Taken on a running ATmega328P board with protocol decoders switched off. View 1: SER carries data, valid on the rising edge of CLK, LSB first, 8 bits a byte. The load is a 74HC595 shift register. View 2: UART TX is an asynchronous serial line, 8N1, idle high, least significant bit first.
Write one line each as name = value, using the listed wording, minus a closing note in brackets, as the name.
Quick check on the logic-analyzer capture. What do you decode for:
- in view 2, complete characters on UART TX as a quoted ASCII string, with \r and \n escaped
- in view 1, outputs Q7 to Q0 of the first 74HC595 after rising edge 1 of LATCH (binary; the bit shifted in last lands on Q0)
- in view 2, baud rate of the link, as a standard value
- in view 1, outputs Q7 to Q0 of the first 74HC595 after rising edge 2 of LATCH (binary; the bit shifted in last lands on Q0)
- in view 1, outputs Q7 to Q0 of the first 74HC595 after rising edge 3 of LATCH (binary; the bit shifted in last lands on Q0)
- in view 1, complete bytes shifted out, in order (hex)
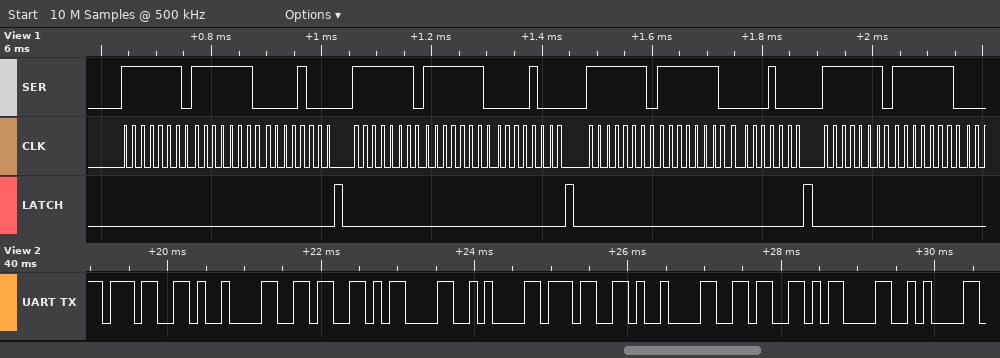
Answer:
in view 2, complete characters on UART TX as a quoted ASCII string, with \r and \n escaped = "7\t6\r\n7\t6\r\n"
in view 1, outputs Q7 to Q0 of the first 74HC595 after rising edge 1 of LATCH = 00001000
in view 2, baud rate of the link, as a standard value = 9600 baud
in view 1, outputs Q7 to Q0 of the first 74HC595 after rising edge 2 of LATCH = 00001000
in view 1, outputs Q7 to Q0 of the first 74HC595 after rising edge 3 of LATCH = 00001000
in view 1, complete bytes shifted out, in order = 7F 7F 10 7F 7F 10 7F 7F 10 7F 7F
